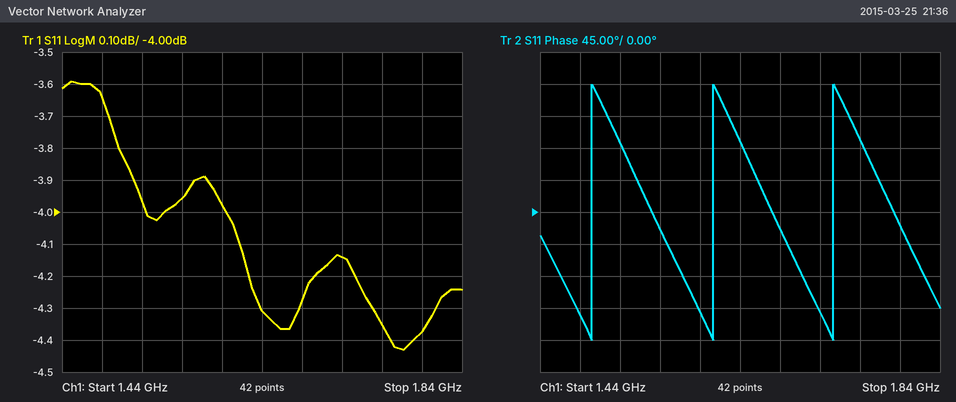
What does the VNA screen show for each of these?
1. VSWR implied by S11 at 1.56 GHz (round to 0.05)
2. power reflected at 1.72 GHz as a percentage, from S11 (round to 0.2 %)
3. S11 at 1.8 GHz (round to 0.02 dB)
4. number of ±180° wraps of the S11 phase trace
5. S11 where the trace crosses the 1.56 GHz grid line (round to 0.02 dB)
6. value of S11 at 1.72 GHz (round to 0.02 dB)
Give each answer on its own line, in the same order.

4.45
38.6 %
-4.38 dB
3
-3.96 dB
-4.14 dB
